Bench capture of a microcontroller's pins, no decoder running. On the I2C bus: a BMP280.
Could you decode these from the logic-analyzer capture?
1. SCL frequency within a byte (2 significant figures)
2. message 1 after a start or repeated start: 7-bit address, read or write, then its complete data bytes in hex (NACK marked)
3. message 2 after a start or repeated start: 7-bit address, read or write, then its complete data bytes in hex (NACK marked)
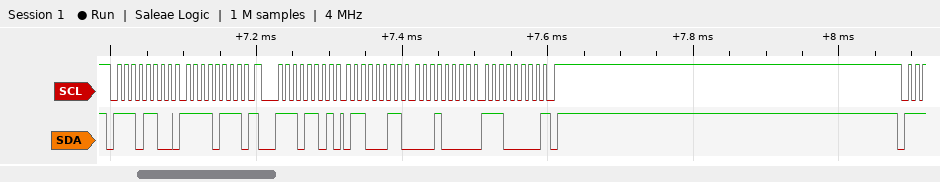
100 kHz
0x76 write: F7
0x76 read: 63 10 E0 NACK
